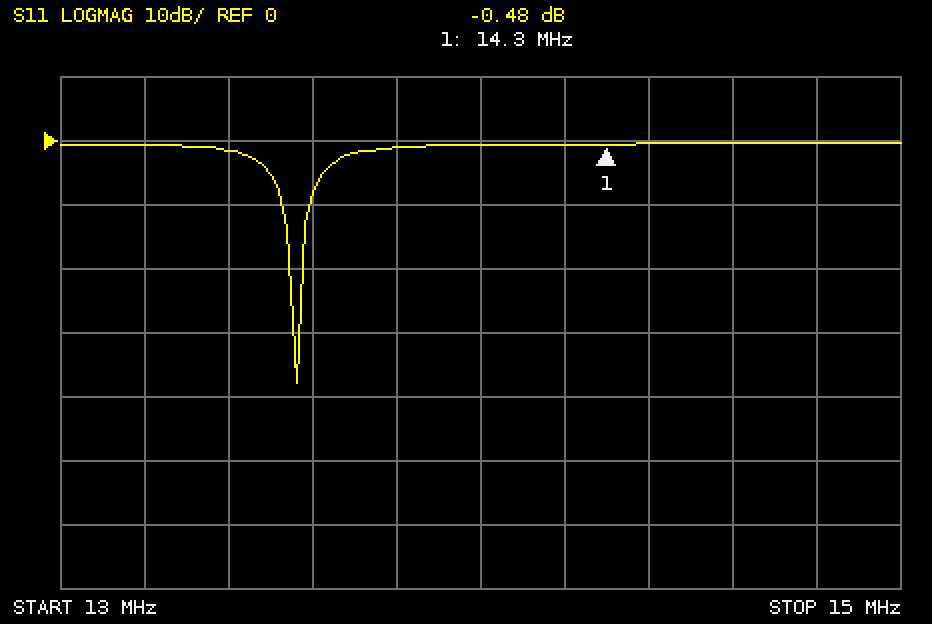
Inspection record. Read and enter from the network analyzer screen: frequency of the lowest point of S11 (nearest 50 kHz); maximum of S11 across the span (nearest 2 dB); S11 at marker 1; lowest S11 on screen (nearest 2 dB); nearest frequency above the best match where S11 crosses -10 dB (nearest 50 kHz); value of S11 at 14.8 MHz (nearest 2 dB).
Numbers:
13.55 MHz
0 dB
-0.48 dB
-38 dB
13.60 MHz
0 dB
